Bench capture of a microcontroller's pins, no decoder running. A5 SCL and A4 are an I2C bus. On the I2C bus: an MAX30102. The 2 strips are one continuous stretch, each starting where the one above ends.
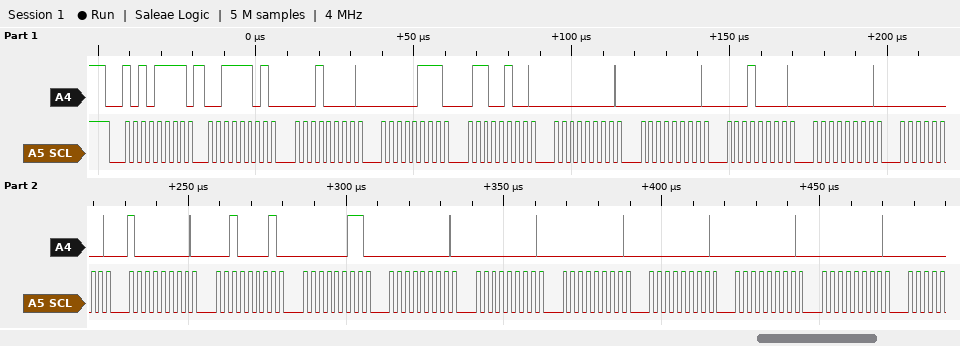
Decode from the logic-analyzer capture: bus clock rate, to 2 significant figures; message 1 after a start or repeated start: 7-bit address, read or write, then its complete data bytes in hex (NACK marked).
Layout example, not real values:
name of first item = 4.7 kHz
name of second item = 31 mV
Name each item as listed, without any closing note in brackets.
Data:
bus clock rate, to 2 significant figures = 400 kHz
message 1 after a start or repeated start: 7-bit address, read or write, then its complete data bytes in hex = 0x57 read: 3D 10 07 64 00 00 10 00 00 80 21 03 00 00 00 00 00 00
